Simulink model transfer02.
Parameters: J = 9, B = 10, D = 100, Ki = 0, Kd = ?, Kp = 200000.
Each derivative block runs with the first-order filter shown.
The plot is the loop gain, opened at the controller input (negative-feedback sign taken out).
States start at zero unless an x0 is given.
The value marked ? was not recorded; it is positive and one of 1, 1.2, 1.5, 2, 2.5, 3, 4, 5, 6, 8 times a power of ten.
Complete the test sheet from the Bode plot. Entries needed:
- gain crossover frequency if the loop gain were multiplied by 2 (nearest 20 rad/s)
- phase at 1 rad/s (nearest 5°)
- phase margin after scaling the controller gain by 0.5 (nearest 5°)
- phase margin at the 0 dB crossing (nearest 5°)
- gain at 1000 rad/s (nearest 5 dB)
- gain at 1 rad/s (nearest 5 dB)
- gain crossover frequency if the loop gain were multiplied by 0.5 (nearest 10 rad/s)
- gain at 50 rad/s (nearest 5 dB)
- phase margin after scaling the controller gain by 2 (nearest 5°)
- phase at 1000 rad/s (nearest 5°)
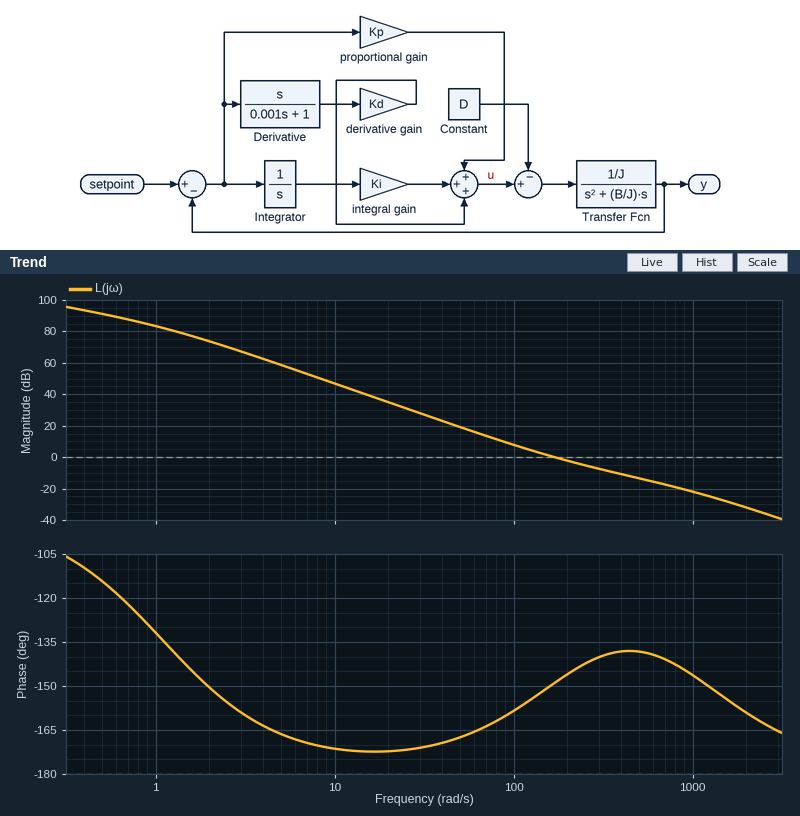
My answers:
260 rad/s
-130°
25°
30°
-20 dB
85 dB
110 rad/s
20 dB
40°
-145°
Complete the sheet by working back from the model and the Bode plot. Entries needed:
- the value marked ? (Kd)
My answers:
800
